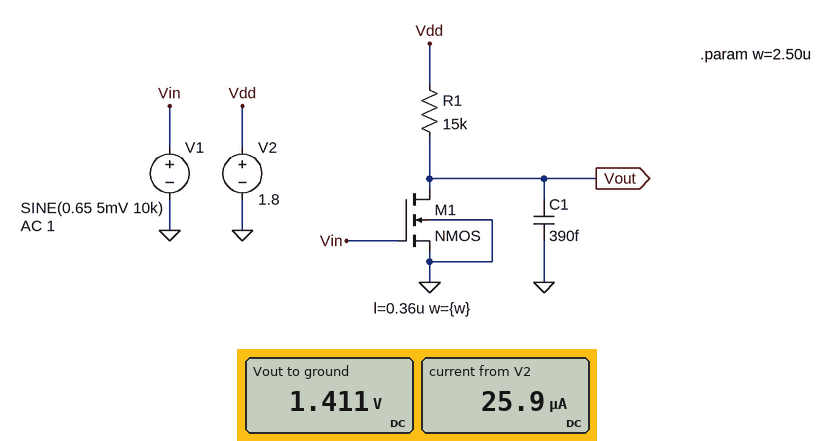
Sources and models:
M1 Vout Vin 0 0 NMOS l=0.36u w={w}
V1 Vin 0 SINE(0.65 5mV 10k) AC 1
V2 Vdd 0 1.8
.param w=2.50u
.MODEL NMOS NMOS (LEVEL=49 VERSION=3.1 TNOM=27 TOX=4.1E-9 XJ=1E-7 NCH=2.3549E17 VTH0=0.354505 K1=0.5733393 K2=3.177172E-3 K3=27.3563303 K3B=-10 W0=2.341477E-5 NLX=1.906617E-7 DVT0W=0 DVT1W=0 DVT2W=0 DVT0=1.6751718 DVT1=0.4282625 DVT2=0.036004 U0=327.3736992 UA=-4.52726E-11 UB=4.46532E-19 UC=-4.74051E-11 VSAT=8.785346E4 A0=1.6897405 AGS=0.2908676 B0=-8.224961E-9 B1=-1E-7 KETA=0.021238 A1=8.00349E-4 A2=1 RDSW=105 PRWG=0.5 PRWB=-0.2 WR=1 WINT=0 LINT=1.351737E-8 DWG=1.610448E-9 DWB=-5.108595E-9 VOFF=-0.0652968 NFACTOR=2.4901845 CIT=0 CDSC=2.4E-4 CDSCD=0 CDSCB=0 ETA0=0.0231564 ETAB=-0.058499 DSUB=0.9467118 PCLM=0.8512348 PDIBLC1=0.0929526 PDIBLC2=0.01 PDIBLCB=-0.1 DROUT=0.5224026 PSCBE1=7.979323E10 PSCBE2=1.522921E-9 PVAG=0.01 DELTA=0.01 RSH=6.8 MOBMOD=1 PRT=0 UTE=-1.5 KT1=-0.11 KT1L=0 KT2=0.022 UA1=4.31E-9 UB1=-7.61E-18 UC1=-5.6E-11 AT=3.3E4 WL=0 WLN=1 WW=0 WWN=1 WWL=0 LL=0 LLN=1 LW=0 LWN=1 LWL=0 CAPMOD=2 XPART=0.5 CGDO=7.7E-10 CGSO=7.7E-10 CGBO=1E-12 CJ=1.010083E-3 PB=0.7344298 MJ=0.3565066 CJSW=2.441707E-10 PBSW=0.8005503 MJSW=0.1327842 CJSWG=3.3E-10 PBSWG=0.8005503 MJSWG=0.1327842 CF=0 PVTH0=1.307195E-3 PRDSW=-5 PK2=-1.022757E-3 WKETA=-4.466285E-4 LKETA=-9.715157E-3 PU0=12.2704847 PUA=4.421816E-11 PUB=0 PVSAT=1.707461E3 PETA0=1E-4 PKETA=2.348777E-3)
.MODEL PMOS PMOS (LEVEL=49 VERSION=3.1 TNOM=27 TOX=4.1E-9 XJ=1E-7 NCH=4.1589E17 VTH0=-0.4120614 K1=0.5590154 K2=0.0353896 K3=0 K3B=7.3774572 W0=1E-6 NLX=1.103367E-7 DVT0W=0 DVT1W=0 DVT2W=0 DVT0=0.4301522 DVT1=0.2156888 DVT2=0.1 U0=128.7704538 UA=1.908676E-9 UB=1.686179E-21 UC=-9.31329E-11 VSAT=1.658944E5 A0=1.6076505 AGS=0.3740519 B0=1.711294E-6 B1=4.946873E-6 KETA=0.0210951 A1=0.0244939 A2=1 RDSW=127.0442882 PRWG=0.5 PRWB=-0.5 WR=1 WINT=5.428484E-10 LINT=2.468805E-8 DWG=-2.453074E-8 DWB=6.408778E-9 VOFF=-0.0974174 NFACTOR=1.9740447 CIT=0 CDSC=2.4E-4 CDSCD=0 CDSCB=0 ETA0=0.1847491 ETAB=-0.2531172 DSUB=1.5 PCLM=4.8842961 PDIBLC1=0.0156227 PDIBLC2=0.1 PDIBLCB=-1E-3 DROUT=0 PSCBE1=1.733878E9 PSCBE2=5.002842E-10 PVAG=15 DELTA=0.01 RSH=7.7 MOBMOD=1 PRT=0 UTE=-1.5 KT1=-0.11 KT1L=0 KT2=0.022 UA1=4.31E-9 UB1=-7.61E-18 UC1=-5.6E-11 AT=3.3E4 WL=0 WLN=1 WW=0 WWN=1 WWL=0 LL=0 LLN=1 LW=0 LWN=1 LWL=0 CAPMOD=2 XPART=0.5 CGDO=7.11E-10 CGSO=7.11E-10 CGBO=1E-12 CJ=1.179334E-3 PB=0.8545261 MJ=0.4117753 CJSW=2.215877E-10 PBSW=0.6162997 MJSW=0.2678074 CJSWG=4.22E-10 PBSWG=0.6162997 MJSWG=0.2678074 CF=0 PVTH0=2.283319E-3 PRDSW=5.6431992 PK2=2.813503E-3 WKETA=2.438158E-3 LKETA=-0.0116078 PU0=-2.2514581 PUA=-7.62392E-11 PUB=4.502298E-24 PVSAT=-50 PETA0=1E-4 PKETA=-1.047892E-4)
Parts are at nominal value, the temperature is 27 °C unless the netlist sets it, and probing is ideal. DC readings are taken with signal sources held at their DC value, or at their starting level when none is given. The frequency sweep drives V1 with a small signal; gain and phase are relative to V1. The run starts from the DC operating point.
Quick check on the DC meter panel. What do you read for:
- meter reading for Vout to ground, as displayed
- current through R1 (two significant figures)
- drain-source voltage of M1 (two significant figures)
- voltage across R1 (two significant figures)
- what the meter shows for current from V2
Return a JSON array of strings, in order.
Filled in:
["1.411 V", "26 µA", "1.4 V", "390 mV", "25.9 µA"]
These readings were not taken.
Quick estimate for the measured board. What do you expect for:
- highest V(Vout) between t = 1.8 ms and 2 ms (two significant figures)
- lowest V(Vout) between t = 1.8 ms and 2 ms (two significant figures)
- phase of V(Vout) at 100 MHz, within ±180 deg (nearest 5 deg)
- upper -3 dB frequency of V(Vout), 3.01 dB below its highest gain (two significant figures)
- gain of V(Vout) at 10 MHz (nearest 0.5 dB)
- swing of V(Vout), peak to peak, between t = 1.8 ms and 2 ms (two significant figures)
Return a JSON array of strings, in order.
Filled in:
["1.4 V", "1.4 V", "105 deg", "28 MHz", "12.5 dB", "45 mV"]
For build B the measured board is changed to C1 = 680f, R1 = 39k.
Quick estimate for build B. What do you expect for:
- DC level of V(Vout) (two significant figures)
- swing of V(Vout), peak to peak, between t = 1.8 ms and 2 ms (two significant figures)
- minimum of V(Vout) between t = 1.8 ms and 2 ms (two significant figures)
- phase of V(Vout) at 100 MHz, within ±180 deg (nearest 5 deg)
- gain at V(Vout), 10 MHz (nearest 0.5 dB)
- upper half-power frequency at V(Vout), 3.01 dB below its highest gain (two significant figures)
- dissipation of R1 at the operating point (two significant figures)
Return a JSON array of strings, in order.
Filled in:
["850 mV", "110 mV", "790 mV", "95 deg", "15.5 dB", "6.6 MHz", "23 µW"]
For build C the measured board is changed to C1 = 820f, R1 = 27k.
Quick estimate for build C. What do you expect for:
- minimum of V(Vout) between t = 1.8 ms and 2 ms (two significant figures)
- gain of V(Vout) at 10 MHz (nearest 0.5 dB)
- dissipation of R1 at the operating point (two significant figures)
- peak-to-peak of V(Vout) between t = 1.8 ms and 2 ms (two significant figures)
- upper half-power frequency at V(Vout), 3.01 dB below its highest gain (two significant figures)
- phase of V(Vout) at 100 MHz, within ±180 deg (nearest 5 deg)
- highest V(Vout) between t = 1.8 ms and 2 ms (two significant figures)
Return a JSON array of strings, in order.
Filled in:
["1.1 V", "13.5 dB", "17 µW", "77 mV", "7.7 MHz", "95 deg", "1.2 V"]
